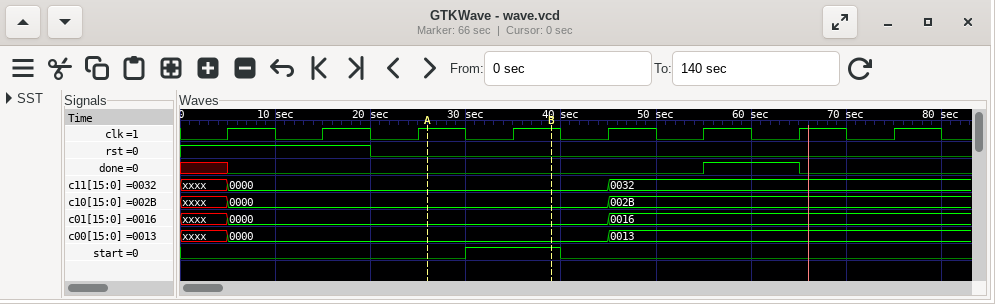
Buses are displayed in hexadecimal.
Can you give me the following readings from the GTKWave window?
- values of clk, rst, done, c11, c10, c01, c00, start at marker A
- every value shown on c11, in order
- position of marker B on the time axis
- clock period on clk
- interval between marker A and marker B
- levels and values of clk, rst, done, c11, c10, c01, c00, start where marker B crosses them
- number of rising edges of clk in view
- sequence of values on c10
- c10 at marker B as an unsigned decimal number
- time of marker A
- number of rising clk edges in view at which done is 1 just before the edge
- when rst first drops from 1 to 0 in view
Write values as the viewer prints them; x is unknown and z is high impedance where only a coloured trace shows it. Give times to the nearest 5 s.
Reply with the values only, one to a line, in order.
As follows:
clk=1, rst=0, done=0, c11=0000, c10=0000, c01=0000, c00=0000, start=0
xxxx, 0000, 0032
40 s
10 s
15 s
clk=1, rst=0, done=0, c11=0000, c10=0000, c01=0000, c00=0000, start=1
8
xxxx, 0000, 002B
0
25 s
1
20 s
